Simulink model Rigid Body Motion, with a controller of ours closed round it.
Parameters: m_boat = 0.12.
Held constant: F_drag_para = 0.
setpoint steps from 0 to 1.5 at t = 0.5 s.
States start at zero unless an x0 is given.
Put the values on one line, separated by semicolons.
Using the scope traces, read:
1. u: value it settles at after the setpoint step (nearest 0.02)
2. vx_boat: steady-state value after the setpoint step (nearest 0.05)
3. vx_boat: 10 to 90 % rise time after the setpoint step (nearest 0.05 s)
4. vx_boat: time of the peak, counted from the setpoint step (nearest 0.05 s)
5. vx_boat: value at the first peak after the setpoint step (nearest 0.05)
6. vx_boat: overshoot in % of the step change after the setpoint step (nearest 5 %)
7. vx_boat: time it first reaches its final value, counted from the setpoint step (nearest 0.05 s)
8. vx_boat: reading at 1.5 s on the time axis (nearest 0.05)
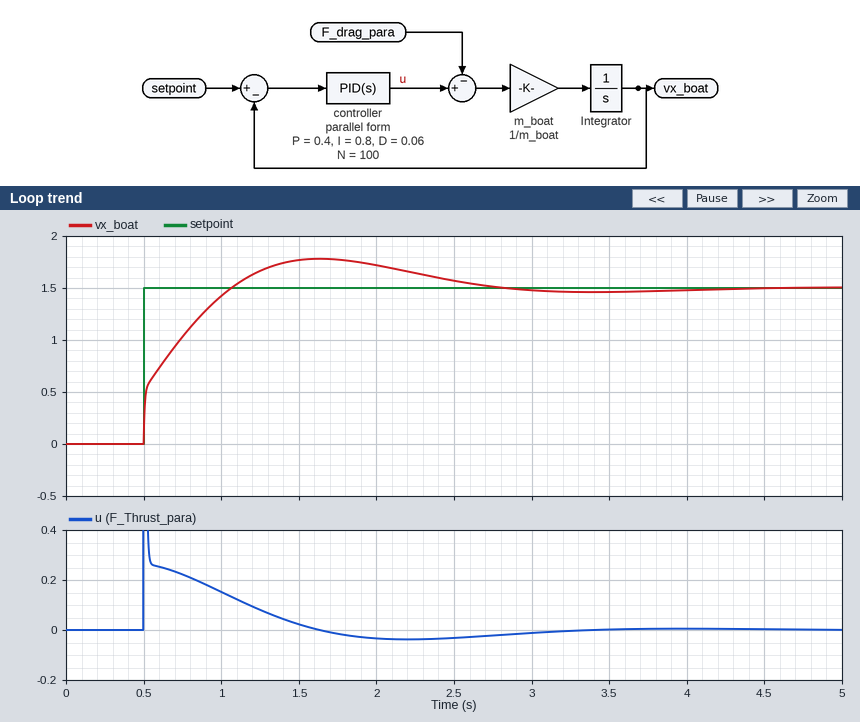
0.00; 1.50; 0.45 s; 1.15 s; 1.80; 20 %; 0.55 s; 1.75
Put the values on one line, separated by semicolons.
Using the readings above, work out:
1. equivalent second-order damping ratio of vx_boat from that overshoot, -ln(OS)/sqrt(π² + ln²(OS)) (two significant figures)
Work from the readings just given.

0.46
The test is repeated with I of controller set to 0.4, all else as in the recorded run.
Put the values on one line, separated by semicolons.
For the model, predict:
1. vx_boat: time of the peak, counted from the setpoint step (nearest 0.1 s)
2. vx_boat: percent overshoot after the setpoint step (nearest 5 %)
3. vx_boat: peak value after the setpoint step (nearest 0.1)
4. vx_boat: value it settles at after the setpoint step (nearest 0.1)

1.5 s; 15 %; 1.7; 1.5
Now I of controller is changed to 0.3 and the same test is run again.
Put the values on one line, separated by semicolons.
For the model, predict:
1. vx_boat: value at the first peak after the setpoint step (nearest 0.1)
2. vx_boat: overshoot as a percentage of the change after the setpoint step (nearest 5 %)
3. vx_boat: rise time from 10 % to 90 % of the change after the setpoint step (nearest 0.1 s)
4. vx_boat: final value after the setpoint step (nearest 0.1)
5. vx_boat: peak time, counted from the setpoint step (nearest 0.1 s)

1.7; 10 %; 0.6 s; 1.5; 1.6 s
